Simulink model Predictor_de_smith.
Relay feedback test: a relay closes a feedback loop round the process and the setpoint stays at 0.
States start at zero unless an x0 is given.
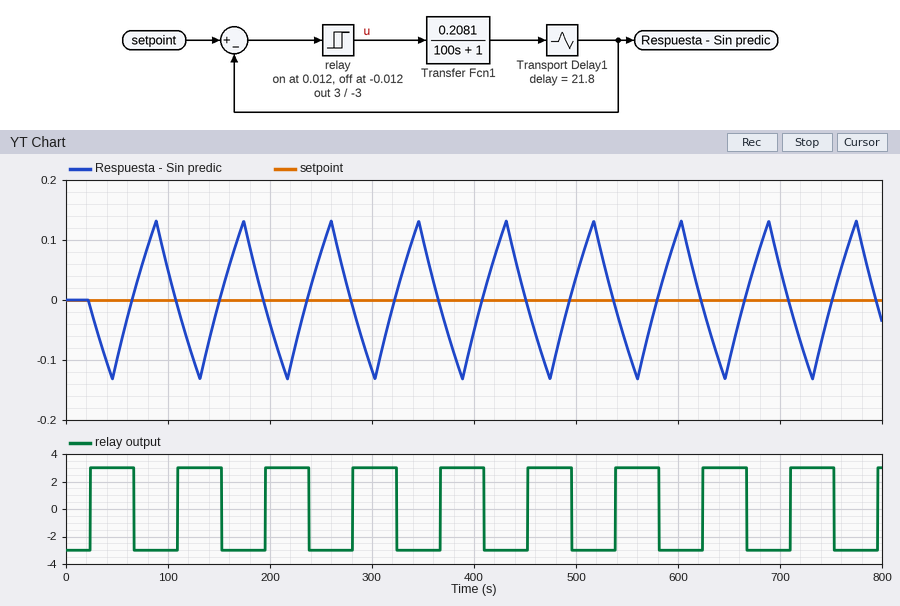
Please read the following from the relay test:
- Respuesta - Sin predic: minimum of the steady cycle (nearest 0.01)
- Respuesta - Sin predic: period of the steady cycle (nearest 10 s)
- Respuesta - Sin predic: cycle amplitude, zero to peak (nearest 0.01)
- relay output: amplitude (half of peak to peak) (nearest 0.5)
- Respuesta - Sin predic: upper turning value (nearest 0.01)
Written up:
-0.13
90 s
0.13
3.0
0.13
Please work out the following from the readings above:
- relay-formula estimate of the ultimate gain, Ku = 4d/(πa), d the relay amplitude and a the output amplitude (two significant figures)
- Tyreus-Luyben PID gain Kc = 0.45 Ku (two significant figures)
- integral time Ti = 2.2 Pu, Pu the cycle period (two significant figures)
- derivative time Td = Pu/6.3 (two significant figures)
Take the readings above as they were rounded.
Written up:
29
13
200 s
14 s
